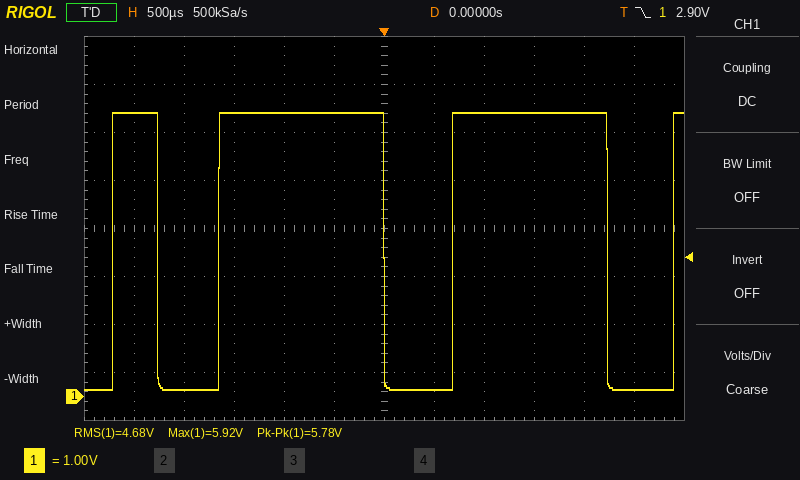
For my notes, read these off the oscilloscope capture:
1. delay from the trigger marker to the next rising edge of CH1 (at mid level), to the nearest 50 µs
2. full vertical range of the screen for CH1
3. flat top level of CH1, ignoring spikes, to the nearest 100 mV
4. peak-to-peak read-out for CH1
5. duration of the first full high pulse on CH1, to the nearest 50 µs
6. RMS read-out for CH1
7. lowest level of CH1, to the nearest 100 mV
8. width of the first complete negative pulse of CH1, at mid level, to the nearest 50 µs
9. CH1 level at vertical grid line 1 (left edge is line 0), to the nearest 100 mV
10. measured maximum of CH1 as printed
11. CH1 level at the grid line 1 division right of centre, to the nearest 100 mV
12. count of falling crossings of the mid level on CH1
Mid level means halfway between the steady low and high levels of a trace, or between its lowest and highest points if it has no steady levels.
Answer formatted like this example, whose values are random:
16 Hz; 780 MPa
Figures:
700 µs; 8 V; 5.9 V; 5.78 V; 450 µs; 4.68 V; 100 mV; 600 µs; 5.9 V; 5.92 V; 100 mV; 3
